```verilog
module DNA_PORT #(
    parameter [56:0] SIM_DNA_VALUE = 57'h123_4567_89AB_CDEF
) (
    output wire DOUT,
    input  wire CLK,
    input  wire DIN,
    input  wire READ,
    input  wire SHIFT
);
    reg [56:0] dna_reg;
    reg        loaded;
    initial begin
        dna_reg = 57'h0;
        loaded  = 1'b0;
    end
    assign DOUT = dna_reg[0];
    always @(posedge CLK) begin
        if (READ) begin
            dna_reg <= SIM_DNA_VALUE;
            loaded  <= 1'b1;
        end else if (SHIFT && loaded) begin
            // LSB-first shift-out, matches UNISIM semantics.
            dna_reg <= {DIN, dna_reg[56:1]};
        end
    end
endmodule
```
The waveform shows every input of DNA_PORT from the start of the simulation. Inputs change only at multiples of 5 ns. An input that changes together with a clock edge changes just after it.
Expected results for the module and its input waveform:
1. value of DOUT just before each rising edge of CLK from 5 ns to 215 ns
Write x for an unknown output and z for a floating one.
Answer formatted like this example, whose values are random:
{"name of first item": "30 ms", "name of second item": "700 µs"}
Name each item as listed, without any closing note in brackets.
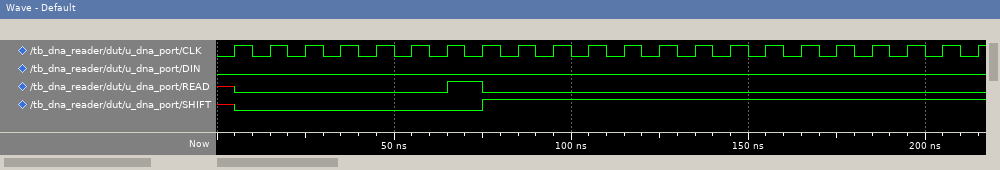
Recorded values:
{"value of DOUT just before each rising edge of CLK from 5 ns to 215 ns": "0 0 0 0 0 0 0 0 1 1 1 1 0 1 1 1 1 0 1 1 0 0"}
